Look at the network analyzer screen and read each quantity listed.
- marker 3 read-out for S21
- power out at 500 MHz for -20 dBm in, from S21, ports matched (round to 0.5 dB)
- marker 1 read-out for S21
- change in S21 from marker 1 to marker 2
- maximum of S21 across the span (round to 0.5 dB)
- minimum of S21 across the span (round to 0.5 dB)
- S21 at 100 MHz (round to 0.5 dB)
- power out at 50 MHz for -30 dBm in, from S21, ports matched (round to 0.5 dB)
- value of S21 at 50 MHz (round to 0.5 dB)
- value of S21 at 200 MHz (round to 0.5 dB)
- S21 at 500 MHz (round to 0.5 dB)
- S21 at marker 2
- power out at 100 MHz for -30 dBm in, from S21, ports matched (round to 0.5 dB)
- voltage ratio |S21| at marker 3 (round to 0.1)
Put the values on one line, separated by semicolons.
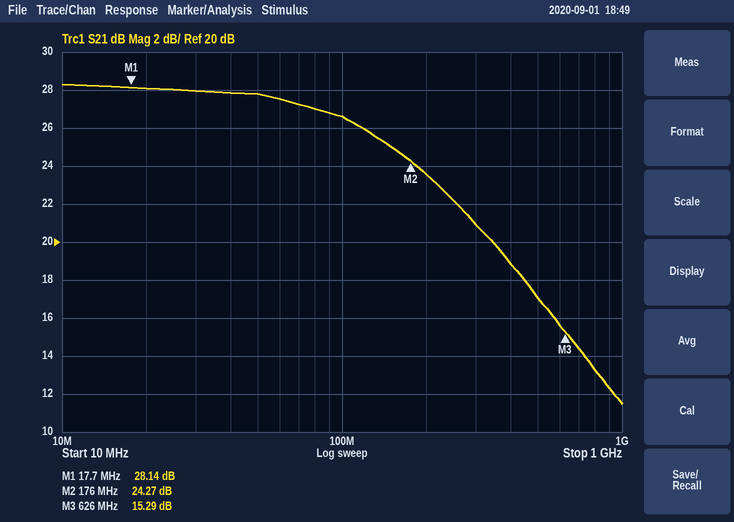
15.29 dB; -3.0 dBm; 28.14 dB; -3.87 dB; 28.5 dB; 11.5 dB; 26.5 dB; -2.0 dBm; 28.0 dB; 23.5 dB; 17.0 dB; 24.27 dB; -3.5 dBm; 5.8
